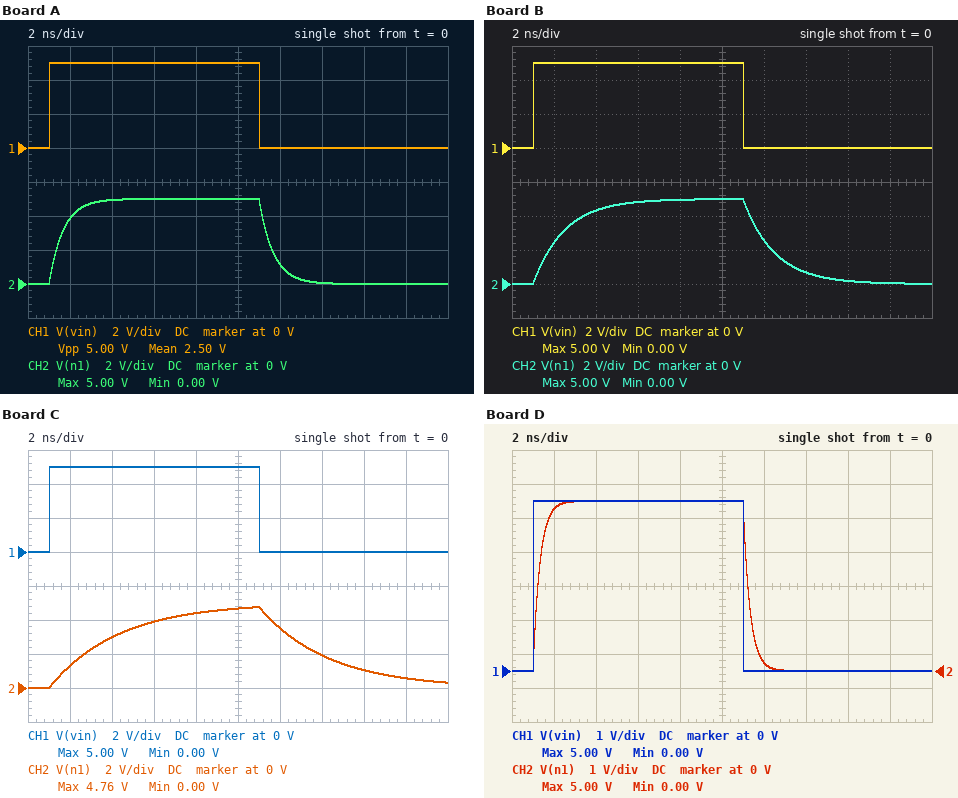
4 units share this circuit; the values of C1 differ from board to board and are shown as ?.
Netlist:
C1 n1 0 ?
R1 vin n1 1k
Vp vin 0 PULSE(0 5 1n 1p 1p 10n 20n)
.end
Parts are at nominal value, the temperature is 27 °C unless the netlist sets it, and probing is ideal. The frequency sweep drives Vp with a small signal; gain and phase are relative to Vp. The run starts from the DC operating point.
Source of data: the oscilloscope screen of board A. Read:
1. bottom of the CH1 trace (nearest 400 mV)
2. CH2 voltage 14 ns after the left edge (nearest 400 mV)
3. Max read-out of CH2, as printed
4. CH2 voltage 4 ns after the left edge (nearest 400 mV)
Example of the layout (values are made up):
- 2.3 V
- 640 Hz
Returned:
- 0 V
- 0 V
- 5.00 V
- 4.8 V
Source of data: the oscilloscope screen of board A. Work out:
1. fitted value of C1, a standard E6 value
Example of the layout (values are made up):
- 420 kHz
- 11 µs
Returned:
- 680 fF
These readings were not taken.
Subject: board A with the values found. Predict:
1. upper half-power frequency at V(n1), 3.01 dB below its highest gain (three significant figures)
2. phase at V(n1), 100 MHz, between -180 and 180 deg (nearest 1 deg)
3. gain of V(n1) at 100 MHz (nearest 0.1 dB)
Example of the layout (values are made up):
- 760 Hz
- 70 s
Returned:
- 234 MHz
- -23 deg
- -0.7 dB
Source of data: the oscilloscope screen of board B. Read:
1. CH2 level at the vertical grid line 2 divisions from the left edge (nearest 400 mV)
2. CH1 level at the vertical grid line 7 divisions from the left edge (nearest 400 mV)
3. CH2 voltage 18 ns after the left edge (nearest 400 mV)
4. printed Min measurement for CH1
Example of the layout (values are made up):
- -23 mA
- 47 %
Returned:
- 4.4 V
- 0 V
- 0 V
- 0.00 V
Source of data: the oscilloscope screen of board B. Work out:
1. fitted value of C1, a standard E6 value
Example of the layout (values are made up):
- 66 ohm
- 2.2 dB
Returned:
- 1.5 pF
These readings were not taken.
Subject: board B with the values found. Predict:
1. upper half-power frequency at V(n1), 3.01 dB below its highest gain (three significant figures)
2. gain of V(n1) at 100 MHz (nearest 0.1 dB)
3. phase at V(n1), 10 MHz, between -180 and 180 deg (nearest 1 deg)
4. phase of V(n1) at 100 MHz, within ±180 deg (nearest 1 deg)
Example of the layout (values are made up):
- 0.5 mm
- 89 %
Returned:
- 106 MHz
- -2.8 dB
- -5 deg
- -43 deg
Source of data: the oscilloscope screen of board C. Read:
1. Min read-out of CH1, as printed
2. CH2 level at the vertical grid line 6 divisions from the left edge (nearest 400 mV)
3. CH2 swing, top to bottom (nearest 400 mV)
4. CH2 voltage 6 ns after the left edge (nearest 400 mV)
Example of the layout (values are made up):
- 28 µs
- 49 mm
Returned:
- 0.00 V
- 3.6 V
- 4.8 V
- 4.0 V
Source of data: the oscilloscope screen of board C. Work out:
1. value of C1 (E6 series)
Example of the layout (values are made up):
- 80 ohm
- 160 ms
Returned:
- 3.3 pF
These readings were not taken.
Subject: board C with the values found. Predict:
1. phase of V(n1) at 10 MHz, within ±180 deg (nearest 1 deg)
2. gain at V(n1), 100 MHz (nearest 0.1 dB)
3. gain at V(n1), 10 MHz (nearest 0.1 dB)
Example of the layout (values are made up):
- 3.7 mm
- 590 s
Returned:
- -12 deg
- -7.2 dB
- -0.2 dB
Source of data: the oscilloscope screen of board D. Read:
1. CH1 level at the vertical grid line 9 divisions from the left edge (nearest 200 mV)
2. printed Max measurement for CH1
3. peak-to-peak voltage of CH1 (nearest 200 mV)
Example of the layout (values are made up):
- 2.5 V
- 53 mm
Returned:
- 0 V
- 5.00 V
- 5.0 V
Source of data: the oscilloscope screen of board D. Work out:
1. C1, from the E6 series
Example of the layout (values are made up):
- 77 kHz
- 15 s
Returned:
- 330 fF
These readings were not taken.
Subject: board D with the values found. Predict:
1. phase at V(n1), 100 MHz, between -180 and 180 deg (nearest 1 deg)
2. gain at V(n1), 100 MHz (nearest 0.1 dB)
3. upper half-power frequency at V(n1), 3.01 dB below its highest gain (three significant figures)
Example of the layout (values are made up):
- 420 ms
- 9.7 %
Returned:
- -12 deg
- -0.2 dB
- 482 MHz
